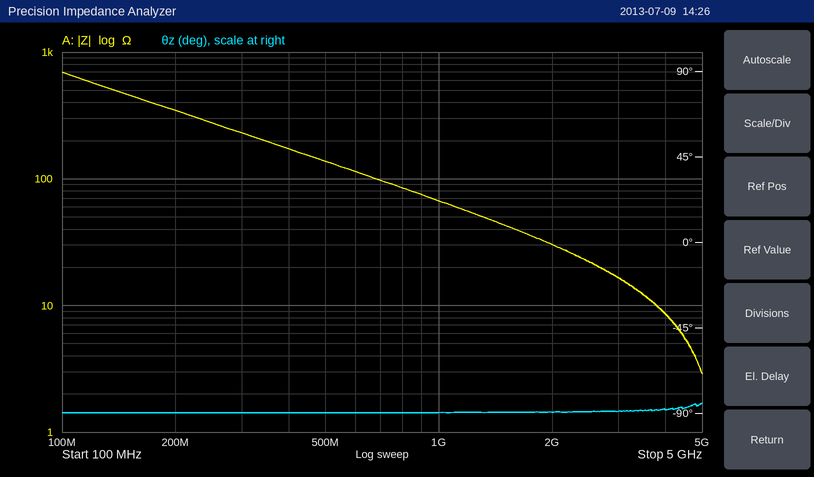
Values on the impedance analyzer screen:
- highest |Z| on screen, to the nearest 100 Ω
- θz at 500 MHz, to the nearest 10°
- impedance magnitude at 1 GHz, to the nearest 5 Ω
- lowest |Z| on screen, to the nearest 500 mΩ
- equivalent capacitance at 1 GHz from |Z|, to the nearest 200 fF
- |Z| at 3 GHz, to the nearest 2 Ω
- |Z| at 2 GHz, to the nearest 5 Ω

700 Ω
-90°
65 Ω
3.0 Ω
2.4 pF
16 Ω
30 Ω
